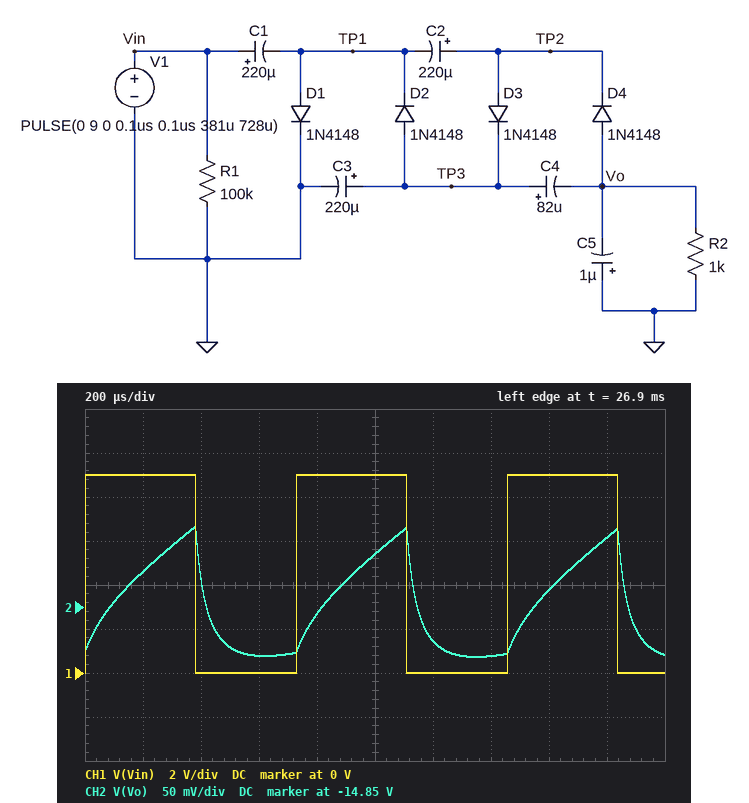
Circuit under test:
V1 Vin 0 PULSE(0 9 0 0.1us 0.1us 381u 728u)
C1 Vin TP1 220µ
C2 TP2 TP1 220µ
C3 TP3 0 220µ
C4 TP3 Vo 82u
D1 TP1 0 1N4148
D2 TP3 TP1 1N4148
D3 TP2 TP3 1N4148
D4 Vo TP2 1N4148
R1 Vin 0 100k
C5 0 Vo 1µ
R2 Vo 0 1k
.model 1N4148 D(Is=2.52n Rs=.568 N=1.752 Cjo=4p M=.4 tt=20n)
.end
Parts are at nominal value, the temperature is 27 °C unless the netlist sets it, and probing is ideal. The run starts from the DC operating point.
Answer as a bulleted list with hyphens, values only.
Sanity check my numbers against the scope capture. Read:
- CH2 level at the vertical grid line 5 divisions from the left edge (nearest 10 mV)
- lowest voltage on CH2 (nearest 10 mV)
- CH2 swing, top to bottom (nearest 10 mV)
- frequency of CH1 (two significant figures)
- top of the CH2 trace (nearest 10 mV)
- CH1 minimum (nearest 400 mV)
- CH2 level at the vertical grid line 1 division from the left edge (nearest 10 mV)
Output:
- -14.79 V
- -14.91 V
- 150 mV
- 1.4 kHz
- -14.76 V
- 0 V
- -14.81 V
